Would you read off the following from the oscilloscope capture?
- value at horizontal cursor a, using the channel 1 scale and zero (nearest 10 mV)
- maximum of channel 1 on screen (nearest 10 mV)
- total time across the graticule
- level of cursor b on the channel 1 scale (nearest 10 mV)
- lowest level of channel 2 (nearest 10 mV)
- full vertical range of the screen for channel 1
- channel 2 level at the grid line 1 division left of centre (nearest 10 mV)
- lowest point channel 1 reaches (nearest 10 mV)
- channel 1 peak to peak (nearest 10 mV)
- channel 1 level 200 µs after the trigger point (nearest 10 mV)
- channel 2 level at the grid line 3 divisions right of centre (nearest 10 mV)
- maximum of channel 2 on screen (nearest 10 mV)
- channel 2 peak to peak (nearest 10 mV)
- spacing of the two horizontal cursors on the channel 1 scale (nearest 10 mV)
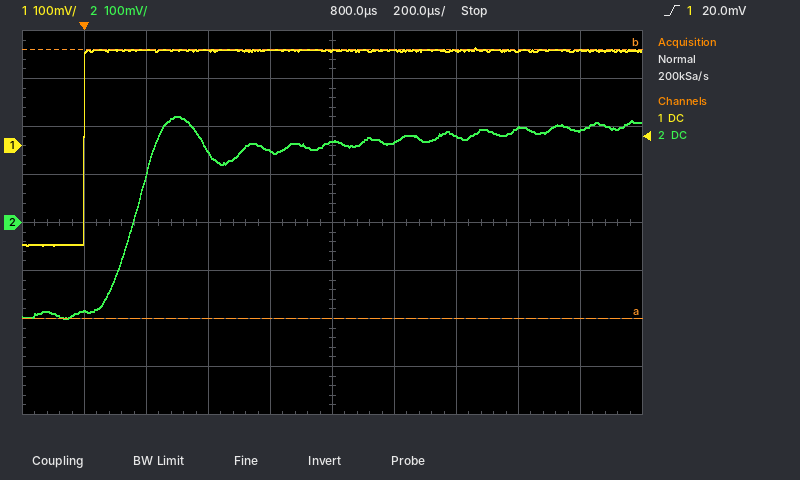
-360 mV
200 mV
2 ms
200 mV
-200 mV
800 mV
150 mV
-210 mV
410 mV
200 mV
200 mV
220 mV
420 mV
560 mV
